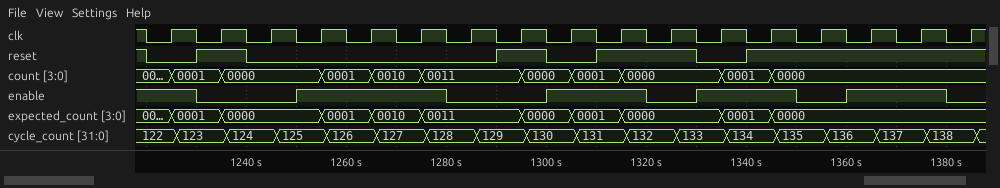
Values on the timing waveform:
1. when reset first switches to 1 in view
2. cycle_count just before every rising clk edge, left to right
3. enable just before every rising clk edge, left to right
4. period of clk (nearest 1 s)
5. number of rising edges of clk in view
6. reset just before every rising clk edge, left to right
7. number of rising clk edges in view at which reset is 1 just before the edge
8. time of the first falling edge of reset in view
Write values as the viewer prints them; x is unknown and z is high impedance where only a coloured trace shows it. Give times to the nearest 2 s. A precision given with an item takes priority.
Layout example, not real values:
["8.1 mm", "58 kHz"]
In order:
["1230 s", "122, 123, 124, 125, 126, 127, 128, 129, 130, 131, 132, 133, 134, 135, 136, 137, 138", "1 0 0 1 1 1 0 0 1 1 0 1 1 0 1 1 0", "10 s", "17", "0 1 0 0 0 0 0 1 0 1 1 0 1 1 1 1 1", "9", "1220 s"]
